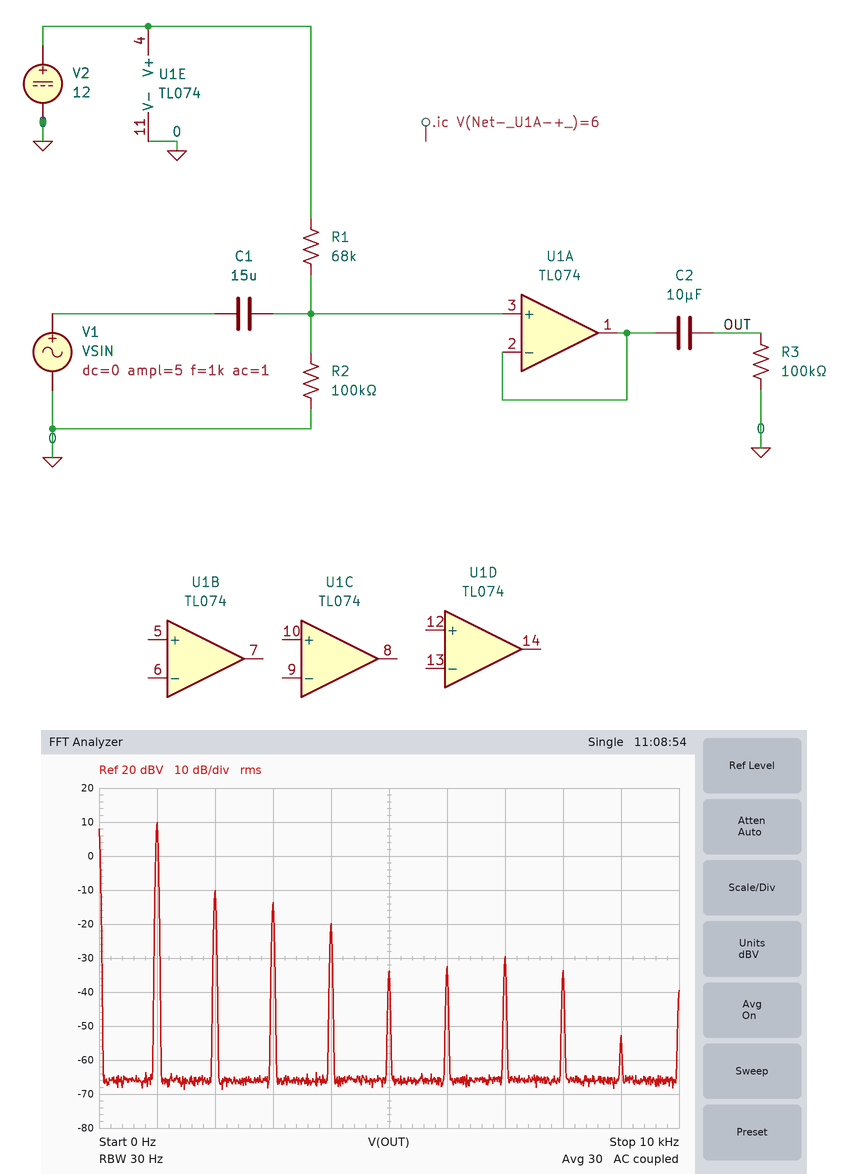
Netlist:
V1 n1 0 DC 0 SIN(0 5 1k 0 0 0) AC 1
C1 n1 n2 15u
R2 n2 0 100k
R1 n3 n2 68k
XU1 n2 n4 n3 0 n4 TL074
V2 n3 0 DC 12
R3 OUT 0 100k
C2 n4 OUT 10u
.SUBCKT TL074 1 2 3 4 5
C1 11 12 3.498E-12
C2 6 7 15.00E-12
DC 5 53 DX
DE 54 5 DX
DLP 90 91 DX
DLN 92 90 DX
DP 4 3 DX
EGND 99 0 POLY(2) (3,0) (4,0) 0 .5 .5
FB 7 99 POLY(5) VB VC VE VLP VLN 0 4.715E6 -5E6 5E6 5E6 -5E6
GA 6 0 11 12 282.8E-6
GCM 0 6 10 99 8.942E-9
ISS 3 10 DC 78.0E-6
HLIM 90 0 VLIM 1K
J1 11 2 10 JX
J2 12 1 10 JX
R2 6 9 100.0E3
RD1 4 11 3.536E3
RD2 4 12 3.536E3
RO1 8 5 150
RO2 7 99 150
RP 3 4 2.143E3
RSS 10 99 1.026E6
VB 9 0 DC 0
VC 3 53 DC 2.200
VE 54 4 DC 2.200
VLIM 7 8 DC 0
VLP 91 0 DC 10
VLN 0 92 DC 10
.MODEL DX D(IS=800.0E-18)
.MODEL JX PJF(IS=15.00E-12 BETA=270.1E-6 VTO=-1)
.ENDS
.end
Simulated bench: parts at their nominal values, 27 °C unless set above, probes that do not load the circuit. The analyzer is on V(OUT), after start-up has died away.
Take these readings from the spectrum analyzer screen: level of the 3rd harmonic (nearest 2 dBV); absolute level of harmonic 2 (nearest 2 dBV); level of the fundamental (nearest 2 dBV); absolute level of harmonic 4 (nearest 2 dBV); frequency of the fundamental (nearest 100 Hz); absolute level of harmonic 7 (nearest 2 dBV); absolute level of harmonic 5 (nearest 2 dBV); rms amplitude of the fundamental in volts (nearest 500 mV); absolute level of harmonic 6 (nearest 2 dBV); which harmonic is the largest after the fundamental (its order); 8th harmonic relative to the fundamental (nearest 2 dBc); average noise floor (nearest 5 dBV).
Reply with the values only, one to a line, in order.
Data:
-14 dBV
-10 dBV
10 dBV
-20 dBV
1.0 kHz
-30 dBV
-34 dBV
3.0 V
-32 dBV
2
-44 dBc
-65 dBV
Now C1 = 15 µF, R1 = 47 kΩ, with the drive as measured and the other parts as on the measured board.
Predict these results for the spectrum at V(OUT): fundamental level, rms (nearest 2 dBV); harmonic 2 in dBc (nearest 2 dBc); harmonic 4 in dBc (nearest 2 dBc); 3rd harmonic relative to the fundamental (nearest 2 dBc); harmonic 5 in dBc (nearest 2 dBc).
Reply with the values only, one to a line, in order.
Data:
8 dBV
-14 dBc
-40 dBc
-22 dBc
-32 dBc
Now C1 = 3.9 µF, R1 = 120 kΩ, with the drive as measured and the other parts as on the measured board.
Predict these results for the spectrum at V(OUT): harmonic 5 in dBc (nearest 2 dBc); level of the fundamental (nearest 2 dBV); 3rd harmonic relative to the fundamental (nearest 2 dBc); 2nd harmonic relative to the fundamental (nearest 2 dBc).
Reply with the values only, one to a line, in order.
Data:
-36 dBc
10 dBV
-28 dBc
-26 dBc
